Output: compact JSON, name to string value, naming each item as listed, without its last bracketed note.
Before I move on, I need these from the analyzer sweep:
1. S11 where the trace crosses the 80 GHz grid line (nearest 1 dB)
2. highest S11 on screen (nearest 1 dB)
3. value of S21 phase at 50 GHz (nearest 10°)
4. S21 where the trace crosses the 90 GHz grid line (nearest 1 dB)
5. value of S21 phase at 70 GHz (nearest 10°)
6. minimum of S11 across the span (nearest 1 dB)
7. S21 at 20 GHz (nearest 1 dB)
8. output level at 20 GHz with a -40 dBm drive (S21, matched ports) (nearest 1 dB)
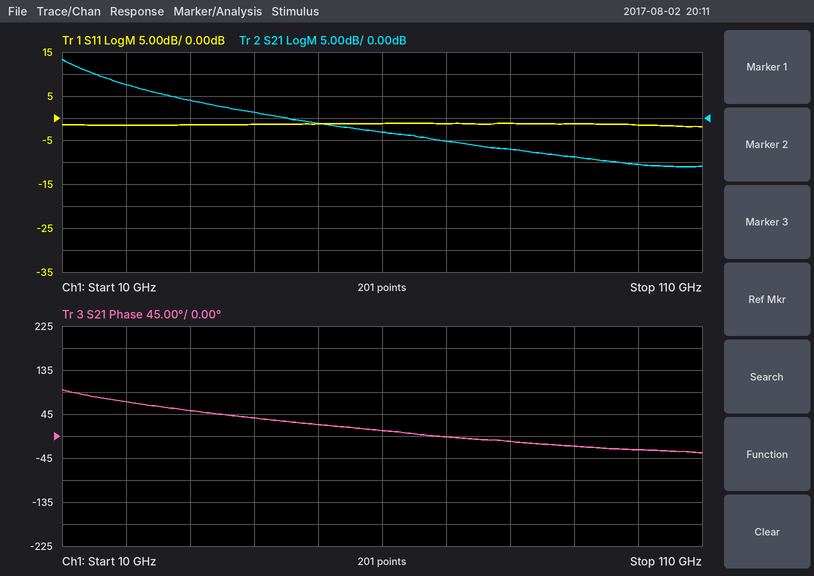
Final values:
{"S11 where the trace crosses the 80 GHz grid line": "-1 dB", "highest S11 on screen": "-1 dB", "value of S21 phase at 50 GHz": "20°", "S21 where the trace crosses the 90 GHz grid line": "-9 dB", "value of S21 phase at 70 GHz": "0°", "minimum of S11 across the span": "-2 dB", "S21 at 20 GHz": "8 dB", "output level at 20 GHz with a -40 dBm drive (S21, matched ports)": "-32 dBm"}
